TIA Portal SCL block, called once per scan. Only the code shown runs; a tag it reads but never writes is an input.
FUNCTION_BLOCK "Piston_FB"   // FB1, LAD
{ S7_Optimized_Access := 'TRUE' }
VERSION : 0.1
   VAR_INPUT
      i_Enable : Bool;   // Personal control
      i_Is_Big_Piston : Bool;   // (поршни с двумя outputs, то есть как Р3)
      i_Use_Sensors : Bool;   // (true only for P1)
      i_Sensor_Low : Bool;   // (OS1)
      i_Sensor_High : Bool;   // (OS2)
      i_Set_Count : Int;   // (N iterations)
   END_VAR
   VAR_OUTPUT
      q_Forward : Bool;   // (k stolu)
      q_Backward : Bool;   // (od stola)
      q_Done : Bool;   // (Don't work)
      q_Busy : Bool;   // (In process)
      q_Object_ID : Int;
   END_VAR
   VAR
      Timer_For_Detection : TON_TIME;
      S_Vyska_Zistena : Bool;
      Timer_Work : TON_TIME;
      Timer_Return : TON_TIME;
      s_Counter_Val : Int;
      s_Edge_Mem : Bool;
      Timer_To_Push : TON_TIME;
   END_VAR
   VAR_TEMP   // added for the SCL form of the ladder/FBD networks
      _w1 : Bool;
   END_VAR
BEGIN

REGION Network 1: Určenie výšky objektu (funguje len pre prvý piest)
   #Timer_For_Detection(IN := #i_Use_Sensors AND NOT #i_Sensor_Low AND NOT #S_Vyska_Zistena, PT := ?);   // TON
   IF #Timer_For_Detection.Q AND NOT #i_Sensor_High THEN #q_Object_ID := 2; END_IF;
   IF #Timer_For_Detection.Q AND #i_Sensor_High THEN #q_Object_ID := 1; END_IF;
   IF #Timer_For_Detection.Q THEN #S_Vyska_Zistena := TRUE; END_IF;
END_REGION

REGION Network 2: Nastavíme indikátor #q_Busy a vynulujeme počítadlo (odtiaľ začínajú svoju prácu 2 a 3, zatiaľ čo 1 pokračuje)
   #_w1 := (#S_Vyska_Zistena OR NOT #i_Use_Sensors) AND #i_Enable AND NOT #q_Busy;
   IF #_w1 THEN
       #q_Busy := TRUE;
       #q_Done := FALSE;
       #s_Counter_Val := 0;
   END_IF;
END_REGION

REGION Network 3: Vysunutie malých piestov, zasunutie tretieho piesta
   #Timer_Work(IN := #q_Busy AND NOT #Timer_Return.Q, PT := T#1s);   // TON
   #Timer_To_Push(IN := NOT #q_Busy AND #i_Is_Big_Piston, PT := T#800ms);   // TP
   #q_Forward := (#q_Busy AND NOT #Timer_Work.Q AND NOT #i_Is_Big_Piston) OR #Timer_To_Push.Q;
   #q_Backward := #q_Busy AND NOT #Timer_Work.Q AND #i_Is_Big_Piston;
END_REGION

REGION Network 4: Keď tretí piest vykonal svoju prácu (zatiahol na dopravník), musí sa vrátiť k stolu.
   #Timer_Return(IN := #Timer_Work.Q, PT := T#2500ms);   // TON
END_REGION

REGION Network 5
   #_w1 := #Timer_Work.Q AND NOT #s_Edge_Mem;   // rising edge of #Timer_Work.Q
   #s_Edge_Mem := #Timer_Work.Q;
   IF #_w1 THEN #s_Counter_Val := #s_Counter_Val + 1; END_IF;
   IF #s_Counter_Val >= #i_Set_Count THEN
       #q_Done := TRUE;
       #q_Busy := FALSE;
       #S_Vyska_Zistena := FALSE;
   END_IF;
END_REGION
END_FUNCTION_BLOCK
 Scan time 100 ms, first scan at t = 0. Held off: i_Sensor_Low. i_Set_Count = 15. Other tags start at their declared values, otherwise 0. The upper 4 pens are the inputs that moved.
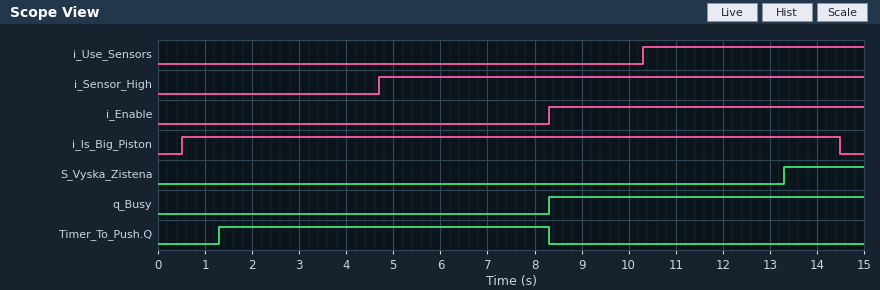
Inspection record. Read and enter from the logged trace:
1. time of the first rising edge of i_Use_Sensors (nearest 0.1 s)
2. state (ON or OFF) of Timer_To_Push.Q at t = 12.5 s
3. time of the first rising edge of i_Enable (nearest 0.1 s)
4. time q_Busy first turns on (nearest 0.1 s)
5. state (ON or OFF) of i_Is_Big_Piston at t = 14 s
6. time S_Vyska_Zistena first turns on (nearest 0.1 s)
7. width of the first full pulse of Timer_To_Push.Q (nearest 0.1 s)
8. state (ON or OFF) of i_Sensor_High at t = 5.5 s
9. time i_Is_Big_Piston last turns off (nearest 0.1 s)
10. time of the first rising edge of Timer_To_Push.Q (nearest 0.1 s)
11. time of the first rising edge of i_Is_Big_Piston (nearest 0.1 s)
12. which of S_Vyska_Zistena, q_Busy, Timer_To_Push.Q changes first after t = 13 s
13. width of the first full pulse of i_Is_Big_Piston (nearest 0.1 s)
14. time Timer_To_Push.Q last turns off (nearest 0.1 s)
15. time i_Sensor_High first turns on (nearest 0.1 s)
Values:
10.3 s
OFF
8.3 s
8.3 s
ON
13.3 s
7.0 s
ON
14.5 s
1.3 s
0.5 s
S_Vyska_Zistena
14.0 s
8.3 s
4.7 s
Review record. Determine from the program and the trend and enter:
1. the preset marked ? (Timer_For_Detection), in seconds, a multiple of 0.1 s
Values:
3.0 s
